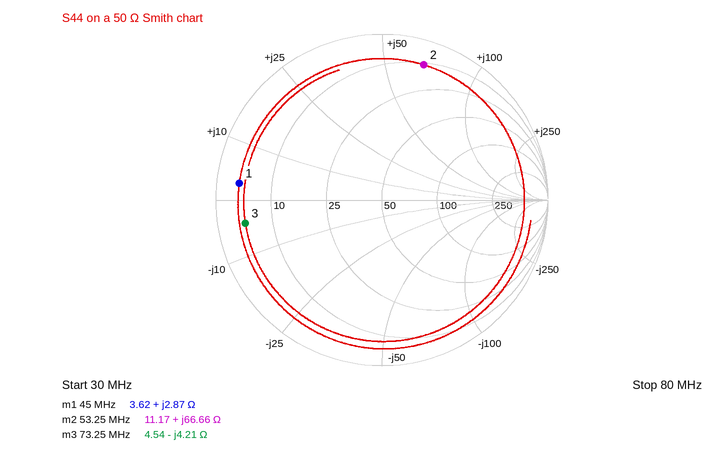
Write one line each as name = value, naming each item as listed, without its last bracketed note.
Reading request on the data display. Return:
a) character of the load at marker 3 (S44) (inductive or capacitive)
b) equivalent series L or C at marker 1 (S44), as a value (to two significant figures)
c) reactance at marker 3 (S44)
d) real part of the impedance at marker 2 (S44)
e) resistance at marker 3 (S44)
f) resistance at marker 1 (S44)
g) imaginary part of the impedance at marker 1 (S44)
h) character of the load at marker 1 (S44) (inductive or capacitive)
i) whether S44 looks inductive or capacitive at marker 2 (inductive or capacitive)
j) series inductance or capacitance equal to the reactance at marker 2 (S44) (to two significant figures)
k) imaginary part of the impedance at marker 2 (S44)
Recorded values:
character of the load at marker 3 (S44) = capacitive
equivalent series L or C at marker 1 (S44), as a value = 10 nH
reactance at marker 3 = -4.21 Ω
real part of the impedance at marker 2 = 11.17 Ω
resistance at marker 3 = 4.54 Ω
resistance at marker 1 = 3.62 Ω
imaginary part of the impedance at marker 1 = +2.87 Ω
character of the load at marker 1 (S44) = inductive
whether S44 looks inductive or capacitive at marker 2 = inductive
series inductance or capacitance equal to the reactance at marker 2 (S44) = 200 nH
imaginary part of the impedance at marker 2 = +66.66 Ω
